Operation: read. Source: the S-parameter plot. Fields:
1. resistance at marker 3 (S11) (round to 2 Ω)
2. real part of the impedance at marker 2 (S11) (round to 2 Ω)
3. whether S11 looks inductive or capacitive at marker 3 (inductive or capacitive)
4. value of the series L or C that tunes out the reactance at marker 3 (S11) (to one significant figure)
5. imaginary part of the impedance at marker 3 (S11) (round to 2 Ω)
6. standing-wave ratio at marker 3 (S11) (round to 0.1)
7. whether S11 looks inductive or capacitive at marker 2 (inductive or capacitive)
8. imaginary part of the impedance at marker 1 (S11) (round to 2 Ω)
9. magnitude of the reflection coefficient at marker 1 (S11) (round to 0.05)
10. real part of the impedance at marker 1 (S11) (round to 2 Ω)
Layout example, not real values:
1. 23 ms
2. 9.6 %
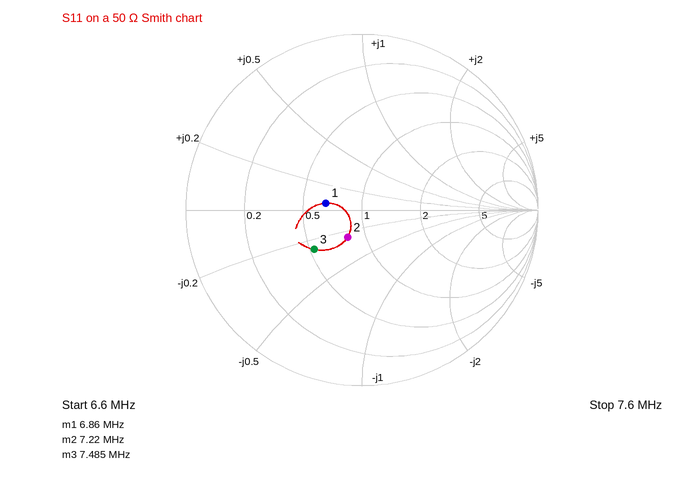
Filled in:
1. 26 Ω
2. 40 Ω
3. capacitive
4. 300 nH
5. -14 Ω
6. 2.1
7. capacitive
8. +2 Ω
9. 0.20
10. 32 Ω
